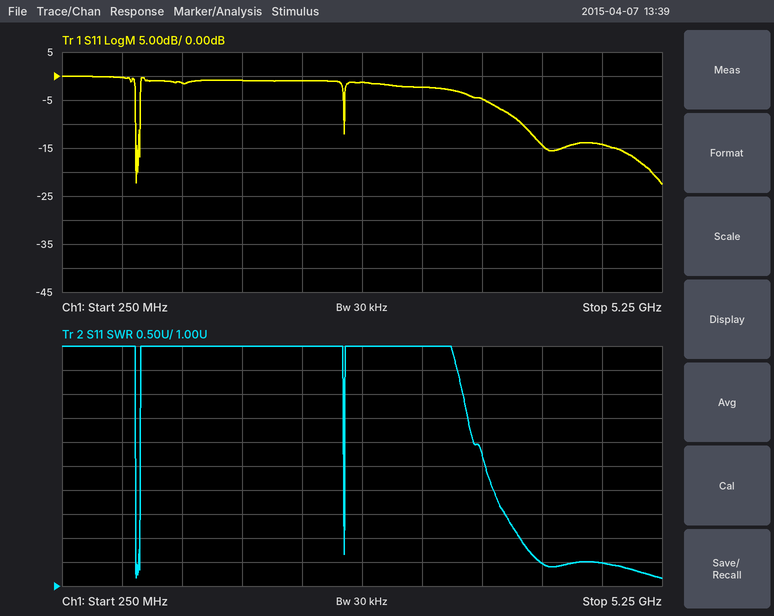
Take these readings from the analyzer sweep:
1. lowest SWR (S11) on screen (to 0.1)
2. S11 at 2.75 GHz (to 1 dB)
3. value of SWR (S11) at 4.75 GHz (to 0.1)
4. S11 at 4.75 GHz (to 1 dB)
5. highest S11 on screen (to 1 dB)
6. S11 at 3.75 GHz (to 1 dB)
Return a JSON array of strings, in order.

["1.2", "-1 dB", "1.5", "-14 dB", "0 dB", "-5 dB"]
